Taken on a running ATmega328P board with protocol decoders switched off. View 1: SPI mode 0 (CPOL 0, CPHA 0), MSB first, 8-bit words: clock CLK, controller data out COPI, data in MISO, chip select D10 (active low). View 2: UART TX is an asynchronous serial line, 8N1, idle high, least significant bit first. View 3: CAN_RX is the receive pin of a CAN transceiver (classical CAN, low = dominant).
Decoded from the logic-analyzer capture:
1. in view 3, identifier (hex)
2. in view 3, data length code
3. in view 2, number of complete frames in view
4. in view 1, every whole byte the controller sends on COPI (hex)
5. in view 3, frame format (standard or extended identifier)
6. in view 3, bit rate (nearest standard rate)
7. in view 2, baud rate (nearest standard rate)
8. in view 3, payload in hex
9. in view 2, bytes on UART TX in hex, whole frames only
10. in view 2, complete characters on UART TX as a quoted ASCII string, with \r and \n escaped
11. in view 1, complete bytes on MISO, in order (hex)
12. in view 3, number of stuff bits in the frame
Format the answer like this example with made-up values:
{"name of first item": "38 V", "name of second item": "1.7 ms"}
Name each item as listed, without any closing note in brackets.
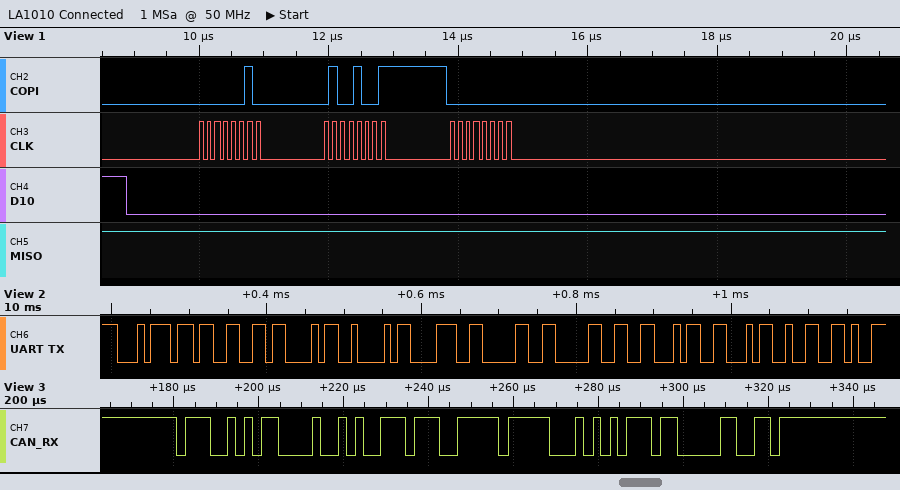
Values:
{"in view 3, identifier": "0x72B", "in view 3, data length code": "4", "in view 2, number of complete frames in view": "10", "in view 1, every whole byte the controller sends on COPI": "0x02 0x49 0x00", "in view 3, frame format": "standard", "in view 3, bit rate": "500 kbit/s", "in view 2, baud rate": "115200 baud", "in view 3, payload in hex": "A7 73 FF 2A", "in view 2, bytes on UART TX in hex, whole frames only": "74 33 43 42 38 30 30 46 46 32", "in view 2, complete characters on UART TX as a quoted ASCII string, with \\r and \\n escaped": "\"t3CB800FF2\"", "in view 1, complete bytes on MISO, in order": "0xFF 0xFF 0xFF", "in view 3, number of stuff bits in the frame": "3"}
